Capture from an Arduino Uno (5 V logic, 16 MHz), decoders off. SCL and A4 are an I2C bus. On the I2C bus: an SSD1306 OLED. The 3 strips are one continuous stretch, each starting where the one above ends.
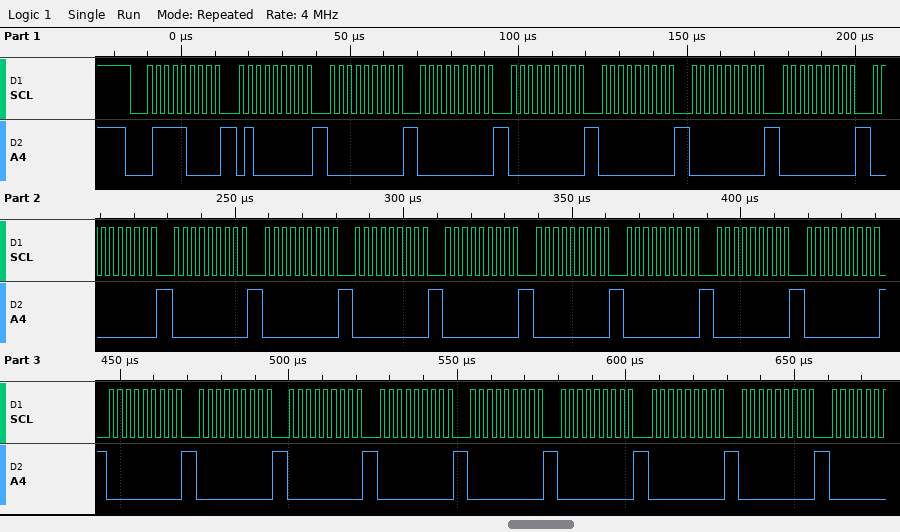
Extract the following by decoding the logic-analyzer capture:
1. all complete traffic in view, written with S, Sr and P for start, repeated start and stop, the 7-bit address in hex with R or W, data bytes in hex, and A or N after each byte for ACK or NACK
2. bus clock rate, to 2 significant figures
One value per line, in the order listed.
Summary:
S 3CW A 40 A 00 A 00 A 00 A 00 A 00 A 00 A 00 A 00 A 00 A 00 A 00 A 00 A 00 A 00 A 00 A 00 A 00 A 00 A 00 A 00 A 00 A 00 A 00 A
400 kHz
